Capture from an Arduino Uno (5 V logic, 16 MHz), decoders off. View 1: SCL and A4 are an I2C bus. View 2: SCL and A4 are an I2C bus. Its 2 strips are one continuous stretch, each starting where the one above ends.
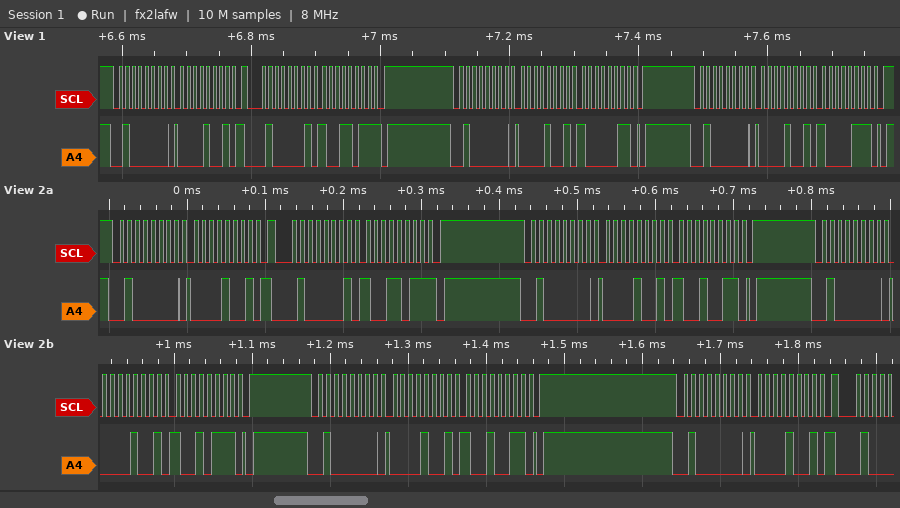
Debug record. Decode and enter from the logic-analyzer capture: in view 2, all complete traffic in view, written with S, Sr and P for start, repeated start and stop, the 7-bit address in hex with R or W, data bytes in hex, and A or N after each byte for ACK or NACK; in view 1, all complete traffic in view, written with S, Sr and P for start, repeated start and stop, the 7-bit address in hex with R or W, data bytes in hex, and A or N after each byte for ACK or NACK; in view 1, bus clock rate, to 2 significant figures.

S 20W A 09 A Sr 20R A 9B N P S 20W A 09 A 93 A P S 20W A 09 A 97 A P S 20W A 09 A 93 A P S 20W A 09 A
S 20W A 09 A Sr 20R A 9B N P S 20W A 09 A 83 A P S 20W A 09 A 87 A P
100 kHz
